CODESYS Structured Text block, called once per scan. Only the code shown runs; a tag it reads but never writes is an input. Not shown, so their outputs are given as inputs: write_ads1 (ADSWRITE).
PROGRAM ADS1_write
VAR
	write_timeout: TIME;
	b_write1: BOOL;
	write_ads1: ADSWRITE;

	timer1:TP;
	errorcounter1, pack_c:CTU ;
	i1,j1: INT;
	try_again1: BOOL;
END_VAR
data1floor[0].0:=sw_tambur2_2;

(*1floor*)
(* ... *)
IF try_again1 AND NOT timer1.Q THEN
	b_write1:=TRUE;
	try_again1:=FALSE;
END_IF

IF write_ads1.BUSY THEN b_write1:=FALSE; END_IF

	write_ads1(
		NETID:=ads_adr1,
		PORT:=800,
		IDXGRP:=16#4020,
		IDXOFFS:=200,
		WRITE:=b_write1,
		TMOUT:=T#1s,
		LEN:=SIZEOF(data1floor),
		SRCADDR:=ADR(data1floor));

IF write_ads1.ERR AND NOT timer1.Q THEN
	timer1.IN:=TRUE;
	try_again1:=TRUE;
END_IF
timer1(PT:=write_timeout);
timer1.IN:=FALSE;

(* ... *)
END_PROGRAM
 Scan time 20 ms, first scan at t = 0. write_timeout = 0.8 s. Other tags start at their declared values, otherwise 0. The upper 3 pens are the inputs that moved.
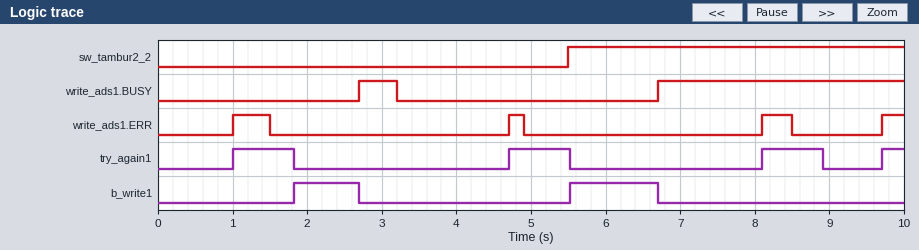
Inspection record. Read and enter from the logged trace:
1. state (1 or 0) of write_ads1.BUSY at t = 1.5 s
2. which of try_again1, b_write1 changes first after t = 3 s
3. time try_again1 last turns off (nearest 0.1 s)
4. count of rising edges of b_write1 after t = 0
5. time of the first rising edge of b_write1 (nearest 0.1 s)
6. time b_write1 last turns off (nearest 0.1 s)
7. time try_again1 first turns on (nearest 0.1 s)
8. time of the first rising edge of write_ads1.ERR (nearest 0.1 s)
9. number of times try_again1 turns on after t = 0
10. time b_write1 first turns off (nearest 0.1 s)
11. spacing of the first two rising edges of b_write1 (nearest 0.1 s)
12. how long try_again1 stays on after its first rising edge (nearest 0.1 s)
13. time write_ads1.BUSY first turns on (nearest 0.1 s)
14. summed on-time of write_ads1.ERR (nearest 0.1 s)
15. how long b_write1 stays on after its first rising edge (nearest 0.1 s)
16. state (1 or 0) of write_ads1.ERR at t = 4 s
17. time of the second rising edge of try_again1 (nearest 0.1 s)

0
try_again1
8.9 s
2
1.8 s
6.7 s
1.0 s
1.0 s
4
2.7 s
3.7 s
0.8 s
2.7 s
1.4 s
0.9 s
0
4.7 s
